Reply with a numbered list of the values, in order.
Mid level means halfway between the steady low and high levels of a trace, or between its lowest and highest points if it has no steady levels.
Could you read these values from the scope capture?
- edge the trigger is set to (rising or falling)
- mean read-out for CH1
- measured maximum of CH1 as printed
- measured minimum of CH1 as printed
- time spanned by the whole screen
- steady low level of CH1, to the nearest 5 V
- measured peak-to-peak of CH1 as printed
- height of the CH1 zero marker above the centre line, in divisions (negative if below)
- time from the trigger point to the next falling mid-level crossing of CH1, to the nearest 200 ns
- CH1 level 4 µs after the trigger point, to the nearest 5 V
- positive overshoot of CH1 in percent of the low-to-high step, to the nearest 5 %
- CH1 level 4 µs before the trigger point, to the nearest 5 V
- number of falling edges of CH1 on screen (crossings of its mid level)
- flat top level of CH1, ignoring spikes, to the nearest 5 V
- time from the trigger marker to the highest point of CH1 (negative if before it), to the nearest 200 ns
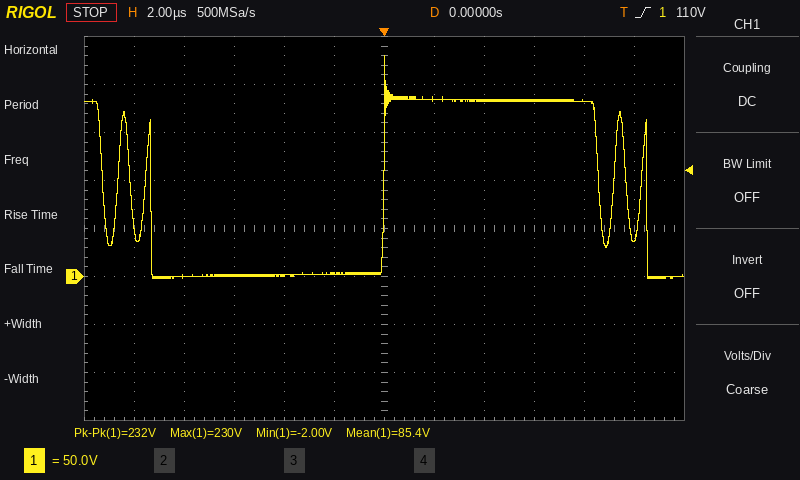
1. rising
2. 85.4 V
3. 230 V
4. -2.00 V
5. 24 µs
6. 0 V
7. 232 V
8. -1.0 div
9. 8.6 µs
10. 185 V
11. 25 %
12. 0 V
13. 6
14. 185 V
15. 0.0 µs
